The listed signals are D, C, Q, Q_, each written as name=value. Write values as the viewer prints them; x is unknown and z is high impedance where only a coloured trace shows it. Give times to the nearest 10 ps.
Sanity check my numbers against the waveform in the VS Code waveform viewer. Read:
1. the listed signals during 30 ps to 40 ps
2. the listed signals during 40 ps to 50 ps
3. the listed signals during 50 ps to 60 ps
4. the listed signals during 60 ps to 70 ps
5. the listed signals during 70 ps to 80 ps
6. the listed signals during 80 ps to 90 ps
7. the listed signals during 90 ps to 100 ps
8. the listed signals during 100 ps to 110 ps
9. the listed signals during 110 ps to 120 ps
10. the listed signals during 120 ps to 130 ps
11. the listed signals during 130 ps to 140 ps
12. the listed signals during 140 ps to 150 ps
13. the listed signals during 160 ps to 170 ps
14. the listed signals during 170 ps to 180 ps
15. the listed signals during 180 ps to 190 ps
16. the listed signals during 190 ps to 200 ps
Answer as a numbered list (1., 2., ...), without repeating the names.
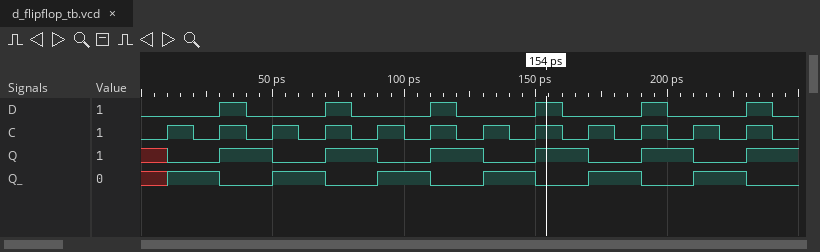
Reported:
1. D=1, C=1, Q=1, Q_=0
2. D=0, C=0, Q=1, Q_=0
3. D=0, C=1, Q=0, Q_=1
4. D=0, C=0, Q=0, Q_=1
5. D=1, C=1, Q=1, Q_=0
6. D=0, C=0, Q=1, Q_=0
7. D=0, C=1, Q=0, Q_=1
8. D=0, C=0, Q=0, Q_=1
9. D=1, C=1, Q=1, Q_=0
10. D=0, C=0, Q=1, Q_=0
11. D=0, C=1, Q=0, Q_=1
12. D=0, C=0, Q=0, Q_=1
13. D=0, C=0, Q=1, Q_=0
14. D=0, C=1, Q=0, Q_=1
15. D=0, C=0, Q=0, Q_=1
16. D=1, C=1, Q=1, Q_=0
